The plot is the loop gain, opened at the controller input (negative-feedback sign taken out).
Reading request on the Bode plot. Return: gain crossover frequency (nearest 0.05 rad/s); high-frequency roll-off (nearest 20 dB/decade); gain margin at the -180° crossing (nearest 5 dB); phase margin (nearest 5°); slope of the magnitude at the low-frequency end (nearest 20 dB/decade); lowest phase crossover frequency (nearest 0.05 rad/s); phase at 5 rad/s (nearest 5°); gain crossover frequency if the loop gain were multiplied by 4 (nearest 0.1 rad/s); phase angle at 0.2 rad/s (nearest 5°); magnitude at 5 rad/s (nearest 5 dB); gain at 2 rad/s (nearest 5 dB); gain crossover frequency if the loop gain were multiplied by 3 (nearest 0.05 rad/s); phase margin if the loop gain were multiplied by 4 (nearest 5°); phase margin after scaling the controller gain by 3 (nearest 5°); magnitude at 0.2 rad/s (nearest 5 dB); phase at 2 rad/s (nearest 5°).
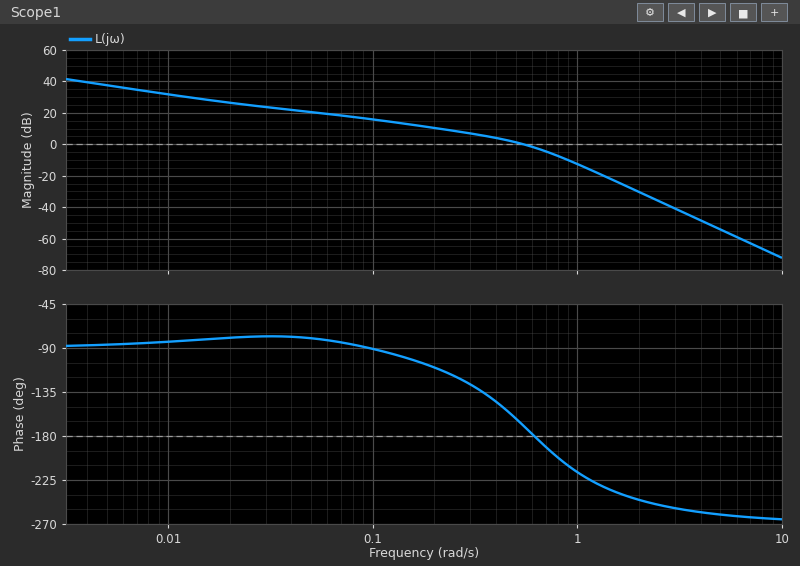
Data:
0.55 rad/s
-60 dB/decade
0 dB
10°
-20 dB/decade
0.60 rad/s
-260°
1.0 rad/s
-110°
-55 dB
-30 dB
0.90 rad/s
-35°
-30°
10 dB
-245°
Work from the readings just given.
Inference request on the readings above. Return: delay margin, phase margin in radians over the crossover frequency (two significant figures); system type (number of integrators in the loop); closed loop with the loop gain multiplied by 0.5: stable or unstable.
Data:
0.32 s
1
stable
